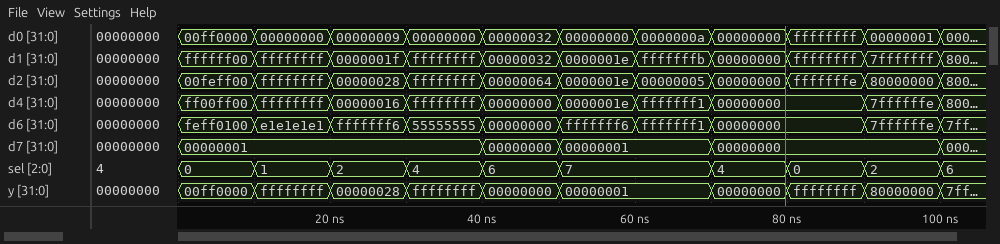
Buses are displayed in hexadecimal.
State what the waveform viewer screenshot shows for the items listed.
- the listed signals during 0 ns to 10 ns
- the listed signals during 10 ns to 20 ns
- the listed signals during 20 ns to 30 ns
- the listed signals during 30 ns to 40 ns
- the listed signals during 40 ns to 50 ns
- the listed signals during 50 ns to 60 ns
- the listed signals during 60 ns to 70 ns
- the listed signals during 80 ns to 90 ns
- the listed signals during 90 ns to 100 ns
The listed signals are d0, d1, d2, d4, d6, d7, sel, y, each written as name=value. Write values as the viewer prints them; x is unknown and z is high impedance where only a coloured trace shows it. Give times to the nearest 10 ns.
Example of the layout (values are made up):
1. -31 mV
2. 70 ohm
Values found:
1. d0=00ff0000, d1=ffffff00, d2=00feff00, d4=ff00ff00, d6=feff0100, d7=00000001, sel=0, y=00ff0000
2. d0=00000000, d1=ffffffff, d2=ffffffff, d4=ffffffff, d6=e1e1e1e1, d7=00000001, sel=1, y=ffffffff
3. d0=00000009, d1=0000001f, d2=00000028, d4=00000016, d6=fffffff6, d7=00000001, sel=2, y=00000028
4. d0=00000000, d1=ffffffff, d2=ffffffff, d4=ffffffff, d6=55555555, d7=00000001, sel=4, y=ffffffff
5. d0=00000032, d1=00000032, d2=00000064, d4=00000000, d6=00000000, d7=00000000, sel=6, y=00000000
6. d0=00000000, d1=0000001e, d2=0000001e, d4=0000001e, d6=fffffff6, d7=00000001, sel=7, y=00000001
7. d0=0000000a, d1=fffffffb, d2=00000005, d4=fffffff1, d6=fffffff1, d7=00000001, sel=7, y=00000001
8. d0=ffffffff, d1=ffffffff, d2=fffffffe, d4=00000000, d6=00000000, d7=00000000, sel=0, y=ffffffff
9. d0=00000001, d1=7fffffff, d2=80000000, d4=7ffffffe, d6=7ffffffe, d7=00000000, sel=2, y=80000000
